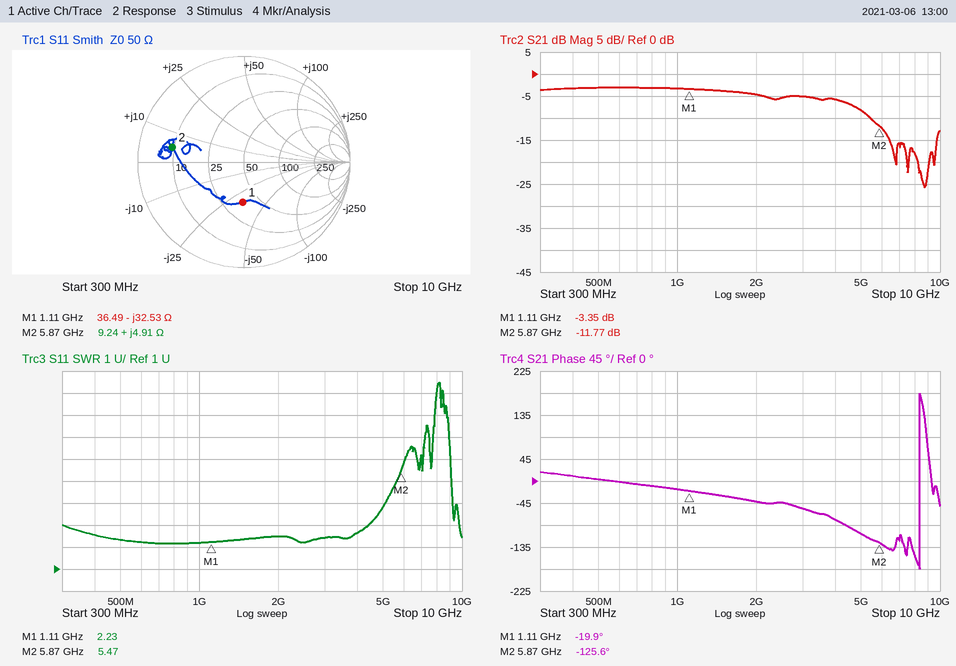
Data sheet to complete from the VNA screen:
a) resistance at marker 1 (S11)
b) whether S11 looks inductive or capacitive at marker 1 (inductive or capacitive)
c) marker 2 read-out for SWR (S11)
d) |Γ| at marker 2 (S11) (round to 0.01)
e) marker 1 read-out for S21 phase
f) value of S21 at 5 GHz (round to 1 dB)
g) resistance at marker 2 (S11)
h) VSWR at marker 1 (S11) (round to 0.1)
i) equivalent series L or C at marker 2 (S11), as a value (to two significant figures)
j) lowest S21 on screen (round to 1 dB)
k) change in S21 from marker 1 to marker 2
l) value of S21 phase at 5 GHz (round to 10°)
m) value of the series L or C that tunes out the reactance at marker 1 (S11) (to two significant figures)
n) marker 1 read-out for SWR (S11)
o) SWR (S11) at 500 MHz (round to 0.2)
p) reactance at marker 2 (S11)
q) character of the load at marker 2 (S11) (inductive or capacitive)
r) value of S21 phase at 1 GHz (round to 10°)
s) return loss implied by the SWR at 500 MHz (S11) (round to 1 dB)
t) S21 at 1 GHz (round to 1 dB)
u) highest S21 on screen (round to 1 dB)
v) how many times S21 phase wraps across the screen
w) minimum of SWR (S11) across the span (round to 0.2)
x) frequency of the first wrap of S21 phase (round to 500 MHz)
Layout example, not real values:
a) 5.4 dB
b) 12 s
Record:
a) 36.49 Ω
b) capacitive
c) 5.47
d) 0.69
e) -19.9°
f) -8 dB
g) 9.24 Ω
h) 2.2
i) 130 pH
j) -26 dB
k) -8.42 dB
l) -110°
m) 4.7 nH
n) 2.23
o) 2.4
p) +4.91 Ω
q) inductive
r) -20°
s) 8 dB
t) -3 dB
u) -3 dB
v) 1
w) 2.2
x) 8.5 GHz
